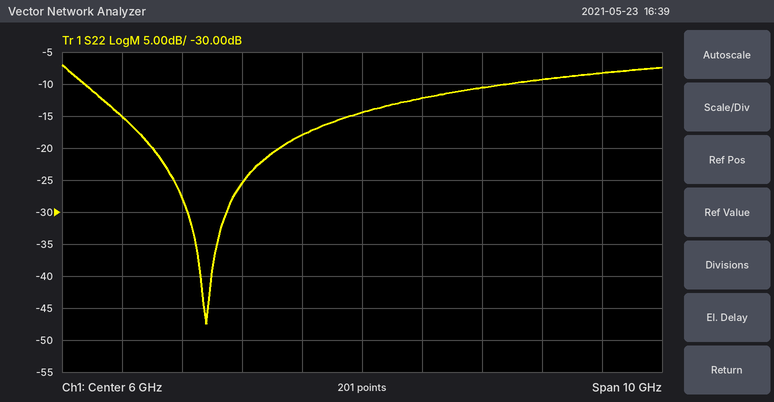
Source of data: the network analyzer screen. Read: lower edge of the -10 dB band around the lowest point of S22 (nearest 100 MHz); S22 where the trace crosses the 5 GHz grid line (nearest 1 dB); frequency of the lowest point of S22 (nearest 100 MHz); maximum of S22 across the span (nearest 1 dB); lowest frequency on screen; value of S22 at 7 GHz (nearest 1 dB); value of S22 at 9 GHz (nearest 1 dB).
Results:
1.4 GHz
-18 dB
3.4 GHz
-7 dB
1 GHz
-12 dB
-9 dB
